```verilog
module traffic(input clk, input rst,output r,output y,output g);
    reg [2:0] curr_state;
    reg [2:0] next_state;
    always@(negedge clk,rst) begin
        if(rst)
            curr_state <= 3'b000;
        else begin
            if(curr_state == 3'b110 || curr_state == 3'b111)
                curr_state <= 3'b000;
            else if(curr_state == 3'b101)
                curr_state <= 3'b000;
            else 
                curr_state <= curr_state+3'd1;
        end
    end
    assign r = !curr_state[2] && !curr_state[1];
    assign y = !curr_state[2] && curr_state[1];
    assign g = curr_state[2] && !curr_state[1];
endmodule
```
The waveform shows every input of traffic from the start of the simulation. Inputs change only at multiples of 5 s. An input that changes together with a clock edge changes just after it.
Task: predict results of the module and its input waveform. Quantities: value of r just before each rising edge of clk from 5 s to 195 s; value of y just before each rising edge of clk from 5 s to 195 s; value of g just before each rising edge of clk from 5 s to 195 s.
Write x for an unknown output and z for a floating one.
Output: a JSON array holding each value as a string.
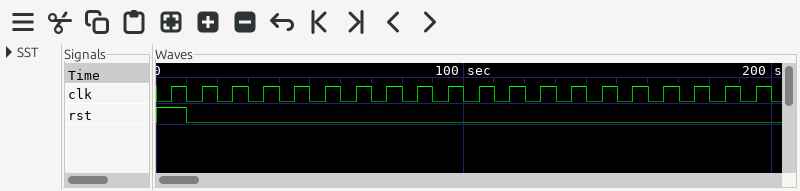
["1 1 0 0 0 0 1 1 0 0 0 0 1 1 0 0 0 0 1 1", "0 0 1 1 0 0 0 0 1 1 0 0 0 0 1 1 0 0 0 0", "0 0 0 0 1 1 0 0 0 0 1 1 0 0 0 0 1 1 0 0"]
